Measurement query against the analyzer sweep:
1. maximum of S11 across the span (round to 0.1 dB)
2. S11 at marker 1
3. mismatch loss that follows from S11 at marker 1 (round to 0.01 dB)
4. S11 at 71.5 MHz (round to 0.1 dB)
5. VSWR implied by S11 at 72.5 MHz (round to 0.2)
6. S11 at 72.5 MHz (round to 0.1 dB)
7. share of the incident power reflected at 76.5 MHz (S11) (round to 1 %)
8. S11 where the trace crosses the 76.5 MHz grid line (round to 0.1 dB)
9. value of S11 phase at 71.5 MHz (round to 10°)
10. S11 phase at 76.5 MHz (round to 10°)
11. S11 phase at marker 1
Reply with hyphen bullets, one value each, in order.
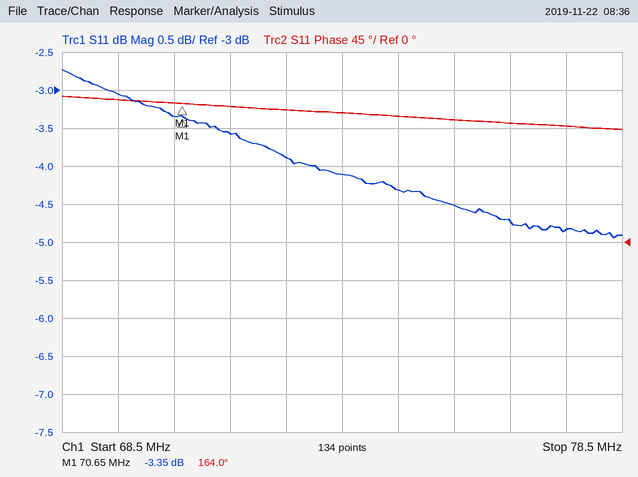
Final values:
- -2.7 dB
- -3.35 dB
- 2.70 dB
- -3.6 dB
- 4.6
- -3.9 dB
- 34 %
- -4.7 dB
- 160°
- 140°
- 164.0°
